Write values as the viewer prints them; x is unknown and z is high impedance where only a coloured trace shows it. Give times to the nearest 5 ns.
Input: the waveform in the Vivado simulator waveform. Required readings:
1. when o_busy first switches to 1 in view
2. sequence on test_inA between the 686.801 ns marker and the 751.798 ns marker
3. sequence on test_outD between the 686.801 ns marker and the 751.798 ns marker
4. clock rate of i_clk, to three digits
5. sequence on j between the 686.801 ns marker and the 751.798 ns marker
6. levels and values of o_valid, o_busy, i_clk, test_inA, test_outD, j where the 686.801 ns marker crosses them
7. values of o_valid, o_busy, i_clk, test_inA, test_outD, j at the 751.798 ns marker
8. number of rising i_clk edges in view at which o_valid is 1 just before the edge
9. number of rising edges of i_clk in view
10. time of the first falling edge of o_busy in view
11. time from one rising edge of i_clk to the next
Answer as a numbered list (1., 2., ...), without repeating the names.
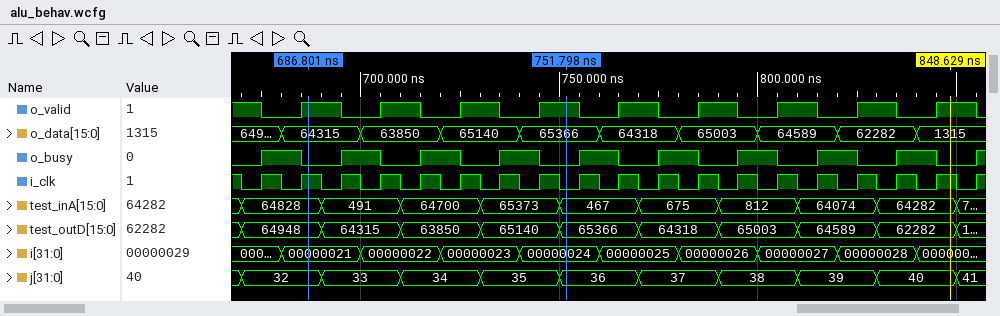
1. 675 ns
2. 64828, 491, 64700, 65373, 467
3. 64948, 64315, 63850, 65140, 65366
4. 100 MHz
5. 32, 33, 34, 35, 36
6. o_valid=1, o_busy=0, i_clk=1, test_inA=64828, test_outD=64948, j=32
7. o_valid=1, o_busy=0, i_clk=0, test_inA=467, test_outD=65366, j=36
8. 10
9. 19
10. 685 ns
11. 10 ns
